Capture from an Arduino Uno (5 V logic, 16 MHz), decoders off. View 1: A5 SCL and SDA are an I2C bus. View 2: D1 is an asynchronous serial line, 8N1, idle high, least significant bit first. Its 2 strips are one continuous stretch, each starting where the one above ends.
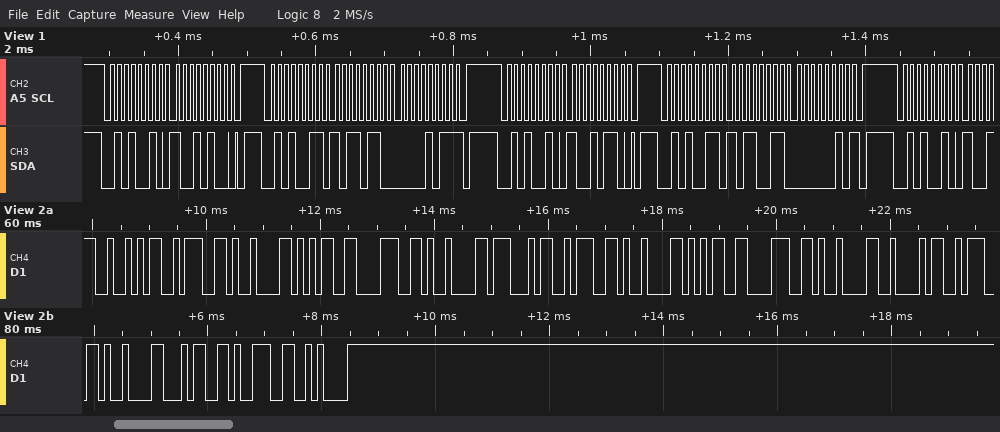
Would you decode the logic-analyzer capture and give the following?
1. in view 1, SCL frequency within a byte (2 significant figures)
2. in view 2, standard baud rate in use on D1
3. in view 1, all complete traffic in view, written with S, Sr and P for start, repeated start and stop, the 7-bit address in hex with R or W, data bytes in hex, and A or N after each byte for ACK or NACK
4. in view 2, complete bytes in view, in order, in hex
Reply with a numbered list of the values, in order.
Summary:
1. 100 kHz
2. 9600 baud
3. S 29W A 94 A P S 29R A B6 A 0B N P S 29W A 96 A P S 29R A B3 A 02 N P S 29W A
4. 0x52 0x3A 0x09 0x35 0x38 0x09 0x47 0x3A 0x09 0x35 0x38 0x09 0x42 0x3A 0x09 0x34 0x39 0x0A
